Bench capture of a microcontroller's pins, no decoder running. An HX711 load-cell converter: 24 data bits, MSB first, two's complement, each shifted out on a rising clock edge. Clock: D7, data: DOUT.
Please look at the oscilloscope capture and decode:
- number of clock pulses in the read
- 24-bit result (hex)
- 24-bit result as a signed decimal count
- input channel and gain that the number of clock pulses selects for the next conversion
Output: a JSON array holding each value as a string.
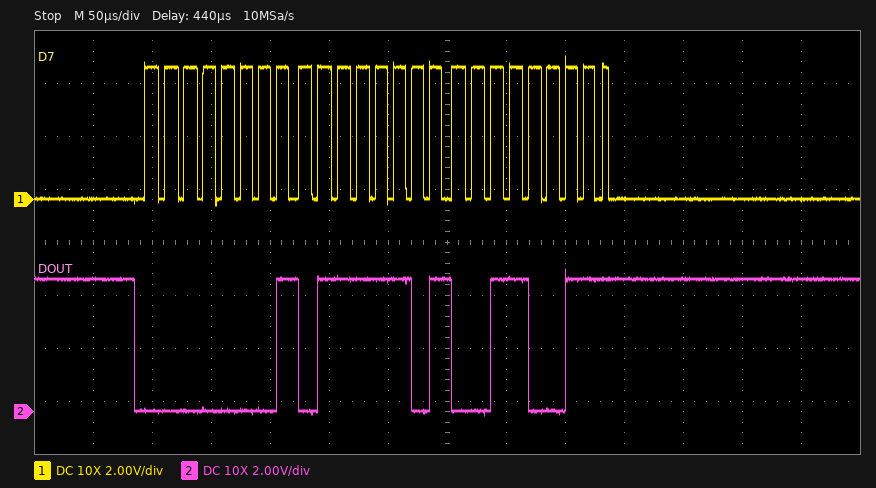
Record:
["25", "0x017D33", "97587", "channel A, gain 128"]
